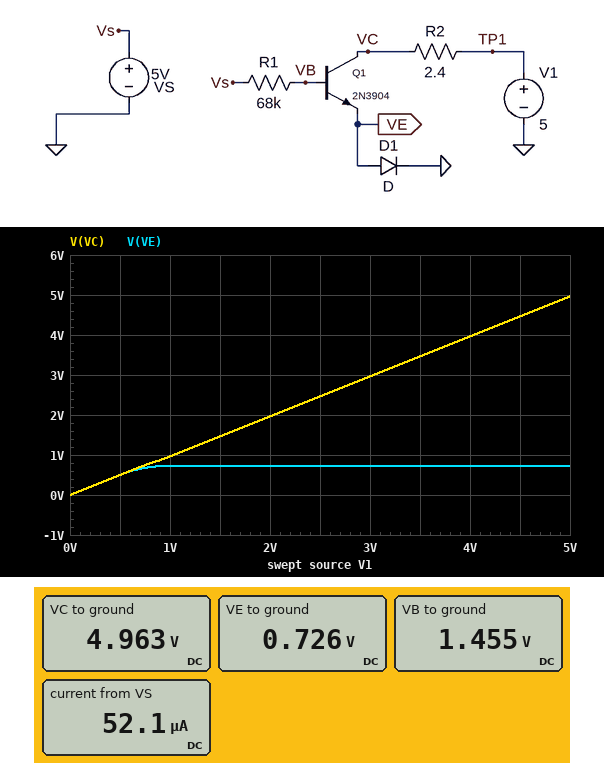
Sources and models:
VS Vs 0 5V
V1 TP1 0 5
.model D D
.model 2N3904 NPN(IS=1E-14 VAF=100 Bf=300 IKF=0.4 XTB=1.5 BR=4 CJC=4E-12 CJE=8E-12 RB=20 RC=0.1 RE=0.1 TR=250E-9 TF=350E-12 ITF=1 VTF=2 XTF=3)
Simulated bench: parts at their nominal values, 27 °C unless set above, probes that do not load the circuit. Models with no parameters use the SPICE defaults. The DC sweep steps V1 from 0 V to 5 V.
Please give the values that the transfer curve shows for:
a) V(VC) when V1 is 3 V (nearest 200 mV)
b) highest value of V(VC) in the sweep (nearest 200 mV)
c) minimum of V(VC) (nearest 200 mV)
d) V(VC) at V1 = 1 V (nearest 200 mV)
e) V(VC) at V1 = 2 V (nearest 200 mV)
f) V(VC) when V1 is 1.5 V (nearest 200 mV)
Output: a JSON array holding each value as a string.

["3.0 V", "5.0 V", "0 V", "1.0 V", "2.0 V", "1.4 V"]
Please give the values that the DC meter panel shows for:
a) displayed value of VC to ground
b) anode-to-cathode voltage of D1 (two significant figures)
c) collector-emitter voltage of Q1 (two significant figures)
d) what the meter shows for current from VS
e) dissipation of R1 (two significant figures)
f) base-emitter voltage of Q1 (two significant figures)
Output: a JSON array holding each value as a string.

["4.963 V", "730 mV", "4.2 V", "52.1 µA", "180 µW", "730 mV"]
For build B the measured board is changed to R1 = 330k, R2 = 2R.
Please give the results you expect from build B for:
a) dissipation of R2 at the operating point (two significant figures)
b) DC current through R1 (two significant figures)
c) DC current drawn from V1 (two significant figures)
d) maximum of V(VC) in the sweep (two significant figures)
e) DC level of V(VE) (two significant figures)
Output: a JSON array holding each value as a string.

["23 µW", "11 µA", "3.4 mA", "5.0 V", "690 mV"]
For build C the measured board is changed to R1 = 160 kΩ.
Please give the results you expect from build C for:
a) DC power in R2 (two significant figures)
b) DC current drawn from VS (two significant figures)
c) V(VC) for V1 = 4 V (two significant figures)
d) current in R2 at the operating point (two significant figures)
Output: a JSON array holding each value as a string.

["110 µW", "22 µA", "4.0 V", "6.9 mA"]
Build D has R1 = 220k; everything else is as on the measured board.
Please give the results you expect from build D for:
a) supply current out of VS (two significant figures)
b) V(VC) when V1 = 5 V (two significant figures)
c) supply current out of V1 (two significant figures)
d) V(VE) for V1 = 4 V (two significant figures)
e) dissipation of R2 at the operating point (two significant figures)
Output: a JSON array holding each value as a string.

["16 µA", "5.0 V", "5.0 mA", "700 mV", "61 µW"]
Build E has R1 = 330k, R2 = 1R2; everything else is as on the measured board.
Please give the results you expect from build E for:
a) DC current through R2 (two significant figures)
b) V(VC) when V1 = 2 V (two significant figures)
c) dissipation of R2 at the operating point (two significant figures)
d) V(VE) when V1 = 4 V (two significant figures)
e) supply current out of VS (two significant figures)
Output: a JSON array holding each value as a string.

["3.4 mA", "2.0 V", "14 µW", "690 mV", "11 µA"]
